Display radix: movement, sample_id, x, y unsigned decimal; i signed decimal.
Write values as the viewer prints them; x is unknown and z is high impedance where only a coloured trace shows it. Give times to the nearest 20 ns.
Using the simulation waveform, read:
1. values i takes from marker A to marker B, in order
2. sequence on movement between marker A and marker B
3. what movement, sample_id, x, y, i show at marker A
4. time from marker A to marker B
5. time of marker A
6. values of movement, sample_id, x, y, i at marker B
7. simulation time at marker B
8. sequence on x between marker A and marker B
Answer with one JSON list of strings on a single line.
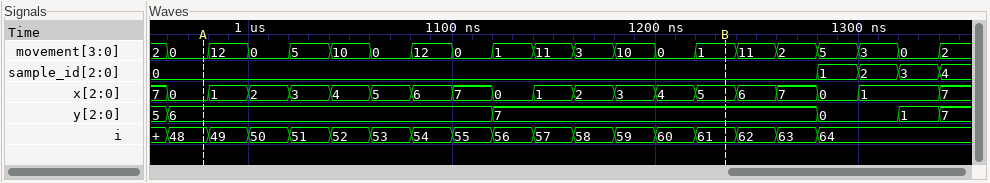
["48, 49, 50, 51, 52, 53, 54, 55, 56, 57, 58, 59, 60, 61", "0, 12, 0, 5, 10, 0, 12, 0, 1, 11, 3, 10, 0, 1", "movement=0, sample_id=0, x=0, y=6, i=48", "260 ns", "980 ns", "movement=1, sample_id=0, x=5, y=7, i=61", "1240 ns", "0, 1, 2, 3, 4, 5, 6, 7, 0, 1, 2, 3, 4, 5"]
